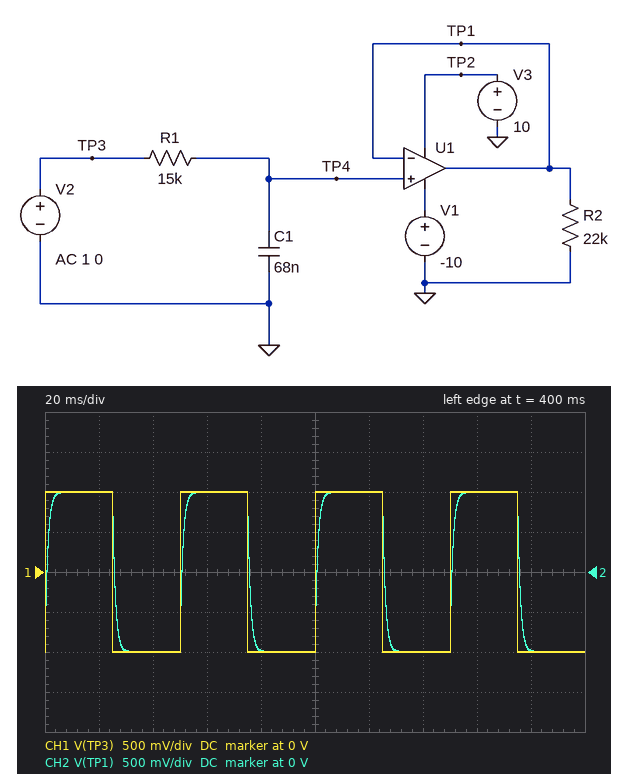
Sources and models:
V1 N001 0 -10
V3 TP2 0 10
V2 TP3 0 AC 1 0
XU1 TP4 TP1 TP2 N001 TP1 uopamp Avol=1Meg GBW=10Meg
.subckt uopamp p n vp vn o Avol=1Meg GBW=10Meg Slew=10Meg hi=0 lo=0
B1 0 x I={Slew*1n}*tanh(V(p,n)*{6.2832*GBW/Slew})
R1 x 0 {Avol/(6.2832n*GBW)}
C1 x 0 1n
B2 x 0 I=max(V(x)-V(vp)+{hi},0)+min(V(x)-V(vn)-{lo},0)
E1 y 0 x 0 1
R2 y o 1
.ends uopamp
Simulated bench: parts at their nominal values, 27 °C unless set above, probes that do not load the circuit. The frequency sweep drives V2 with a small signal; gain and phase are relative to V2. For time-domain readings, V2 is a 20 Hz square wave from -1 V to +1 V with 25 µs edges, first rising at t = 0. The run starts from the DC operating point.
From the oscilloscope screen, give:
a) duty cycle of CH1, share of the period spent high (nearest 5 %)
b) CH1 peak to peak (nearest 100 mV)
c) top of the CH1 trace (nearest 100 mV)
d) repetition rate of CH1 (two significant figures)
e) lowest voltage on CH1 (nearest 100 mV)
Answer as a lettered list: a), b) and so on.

a) 50 %
b) 2.0 V
c) 1.0 V
d) 20 Hz
e) -1.0 V
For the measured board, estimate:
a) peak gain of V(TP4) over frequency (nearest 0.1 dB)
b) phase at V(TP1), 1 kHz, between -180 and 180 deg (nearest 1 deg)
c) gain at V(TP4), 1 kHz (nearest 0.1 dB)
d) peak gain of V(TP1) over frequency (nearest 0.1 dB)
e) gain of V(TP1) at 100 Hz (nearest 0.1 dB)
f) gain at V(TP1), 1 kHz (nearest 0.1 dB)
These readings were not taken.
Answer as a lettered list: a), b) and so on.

a) 0 dB
b) -81 deg
c) -16.2 dB
d) 0 dB
e) -1.5 dB
f) -16.2 dB
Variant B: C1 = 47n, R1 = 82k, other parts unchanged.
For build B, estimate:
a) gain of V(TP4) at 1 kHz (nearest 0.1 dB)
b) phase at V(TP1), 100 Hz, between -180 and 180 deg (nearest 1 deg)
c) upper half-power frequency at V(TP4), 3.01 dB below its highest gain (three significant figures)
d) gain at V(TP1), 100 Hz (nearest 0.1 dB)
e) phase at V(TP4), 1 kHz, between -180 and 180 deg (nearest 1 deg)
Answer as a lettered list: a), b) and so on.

a) -27.7 dB
b) -68 deg
c) 41.3 Hz
d) -8.4 dB
e) -88 deg
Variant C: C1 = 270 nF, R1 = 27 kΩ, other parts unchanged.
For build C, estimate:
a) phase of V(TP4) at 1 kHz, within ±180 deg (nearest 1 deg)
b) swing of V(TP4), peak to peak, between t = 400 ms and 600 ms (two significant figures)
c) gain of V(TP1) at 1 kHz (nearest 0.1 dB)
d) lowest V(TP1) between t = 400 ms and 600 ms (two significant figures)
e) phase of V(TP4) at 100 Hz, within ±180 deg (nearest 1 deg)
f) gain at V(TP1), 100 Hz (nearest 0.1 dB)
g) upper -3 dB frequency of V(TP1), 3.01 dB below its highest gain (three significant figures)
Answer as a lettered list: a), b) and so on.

a) -89 deg
b) 1.9 V
c) -33.2 dB
d) -940 mV
e) -78 deg
f) -13.4 dB
g) 21.8 Hz
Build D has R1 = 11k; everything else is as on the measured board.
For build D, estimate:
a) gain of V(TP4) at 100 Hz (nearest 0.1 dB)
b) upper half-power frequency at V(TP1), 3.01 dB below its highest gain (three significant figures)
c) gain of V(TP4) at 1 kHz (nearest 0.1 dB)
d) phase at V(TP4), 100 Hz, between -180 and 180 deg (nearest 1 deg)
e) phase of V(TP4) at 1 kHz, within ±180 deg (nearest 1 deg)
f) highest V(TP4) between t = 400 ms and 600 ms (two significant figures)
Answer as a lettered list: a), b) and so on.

a) -0.9 dB
b) 213 Hz
c) -13.6 dB
d) -25 deg
e) -78 deg
f) 1.0 V
